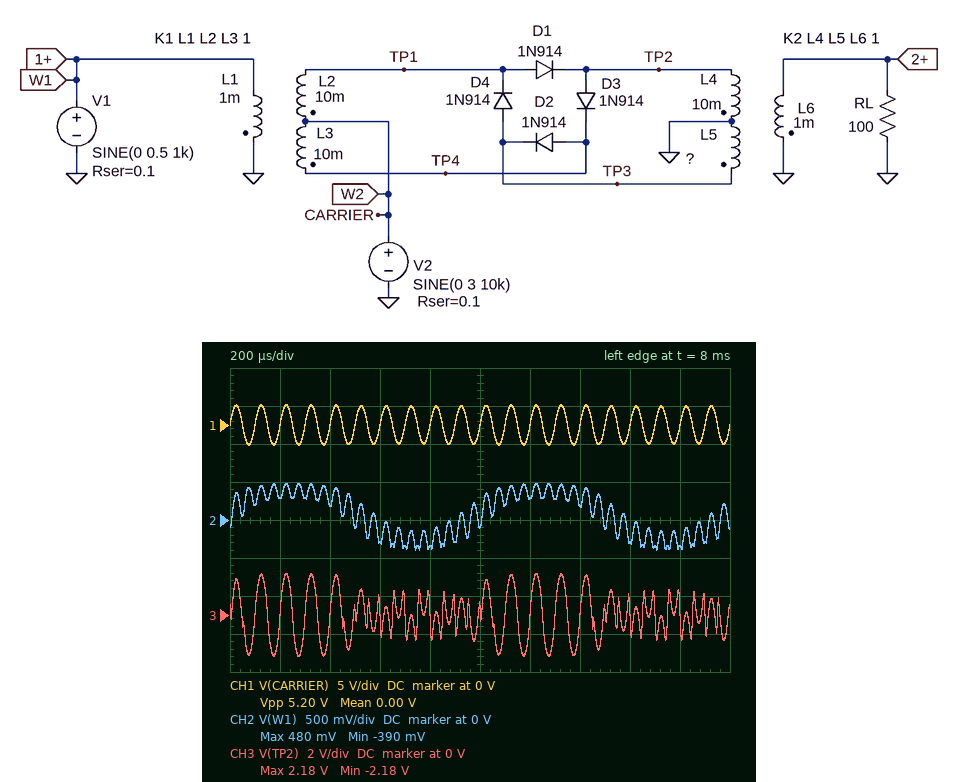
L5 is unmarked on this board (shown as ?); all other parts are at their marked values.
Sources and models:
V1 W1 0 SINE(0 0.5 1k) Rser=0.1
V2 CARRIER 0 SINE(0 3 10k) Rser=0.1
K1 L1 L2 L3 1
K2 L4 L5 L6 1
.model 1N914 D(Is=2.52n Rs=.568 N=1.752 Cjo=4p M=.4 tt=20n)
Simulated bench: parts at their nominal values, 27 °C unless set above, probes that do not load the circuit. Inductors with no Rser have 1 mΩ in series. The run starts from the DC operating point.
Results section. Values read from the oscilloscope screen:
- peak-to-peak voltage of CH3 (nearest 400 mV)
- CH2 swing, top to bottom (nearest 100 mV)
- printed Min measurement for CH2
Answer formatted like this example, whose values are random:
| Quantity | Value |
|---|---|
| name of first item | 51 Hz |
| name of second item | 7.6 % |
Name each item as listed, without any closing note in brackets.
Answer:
| Quantity | Value |
|---|---|
| peak-to-peak voltage of CH3 | 4.4 V |
| CH2 swing, top to bottom | 900 mV |
| printed Min measurement for CH2 | -390 mV |
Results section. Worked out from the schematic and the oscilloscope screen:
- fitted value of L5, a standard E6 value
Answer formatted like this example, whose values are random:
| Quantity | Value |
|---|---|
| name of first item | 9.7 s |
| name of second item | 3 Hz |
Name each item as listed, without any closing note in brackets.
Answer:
| Quantity | Value |
|---|---|
| fitted value of L5, a standard E6 value | 3.3 mH |
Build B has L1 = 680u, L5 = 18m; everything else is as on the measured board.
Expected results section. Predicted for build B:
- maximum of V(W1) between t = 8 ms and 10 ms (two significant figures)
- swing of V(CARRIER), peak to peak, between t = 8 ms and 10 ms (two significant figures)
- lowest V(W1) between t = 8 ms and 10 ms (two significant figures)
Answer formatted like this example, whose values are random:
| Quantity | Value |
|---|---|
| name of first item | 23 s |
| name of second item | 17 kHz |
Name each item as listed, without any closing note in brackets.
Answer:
| Quantity | Value |
|---|---|
| maximum of V(W1) between t = 8 ms and 10 ms | 370 mV |
| swing of V(CARRIER), peak to peak, between t = 8 ms and 10 ms | 5.1 V |
| lowest V(W1) between t = 8 ms and 10 ms | -420 mV |
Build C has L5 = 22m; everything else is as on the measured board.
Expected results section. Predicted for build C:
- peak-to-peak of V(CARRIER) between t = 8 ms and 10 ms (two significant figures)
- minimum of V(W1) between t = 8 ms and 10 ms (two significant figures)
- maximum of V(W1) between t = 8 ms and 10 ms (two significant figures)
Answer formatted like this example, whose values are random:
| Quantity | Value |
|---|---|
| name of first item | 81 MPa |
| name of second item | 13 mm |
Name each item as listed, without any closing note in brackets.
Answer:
| Quantity | Value |
|---|---|
| peak-to-peak of V(CARRIER) between t = 8 ms and 10 ms | 5.1 V |
| minimum of V(W1) between t = 8 ms and 10 ms | -490 mV |
| maximum of V(W1) between t = 8 ms and 10 ms | 400 mV |
